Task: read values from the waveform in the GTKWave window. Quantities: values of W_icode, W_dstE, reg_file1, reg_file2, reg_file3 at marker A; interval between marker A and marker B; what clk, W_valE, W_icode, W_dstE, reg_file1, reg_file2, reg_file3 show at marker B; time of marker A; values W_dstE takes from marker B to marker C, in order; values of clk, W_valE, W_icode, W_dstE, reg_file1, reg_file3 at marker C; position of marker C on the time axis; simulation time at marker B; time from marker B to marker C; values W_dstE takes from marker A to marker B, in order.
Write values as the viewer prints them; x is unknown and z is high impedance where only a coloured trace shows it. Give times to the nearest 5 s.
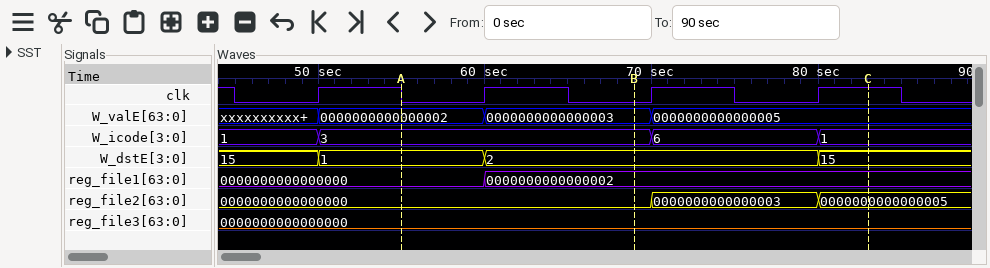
W_icode=3, W_dstE=1, reg_file1=0000000000000000, reg_file2=0000000000000000, reg_file3=0000000000000000
15 s
clk=0, W_valE=0000000000000003, W_icode=3, W_dstE=2, reg_file1=0000000000000002, reg_file2=0000000000000000, reg_file3=0000000000000000
55 s
2, 15
clk=1, W_valE=0000000000000005, W_icode=1, W_dstE=15, reg_file1=0000000000000002, reg_file3=0000000000000000
85 s
70 s
15 s
1, 2
